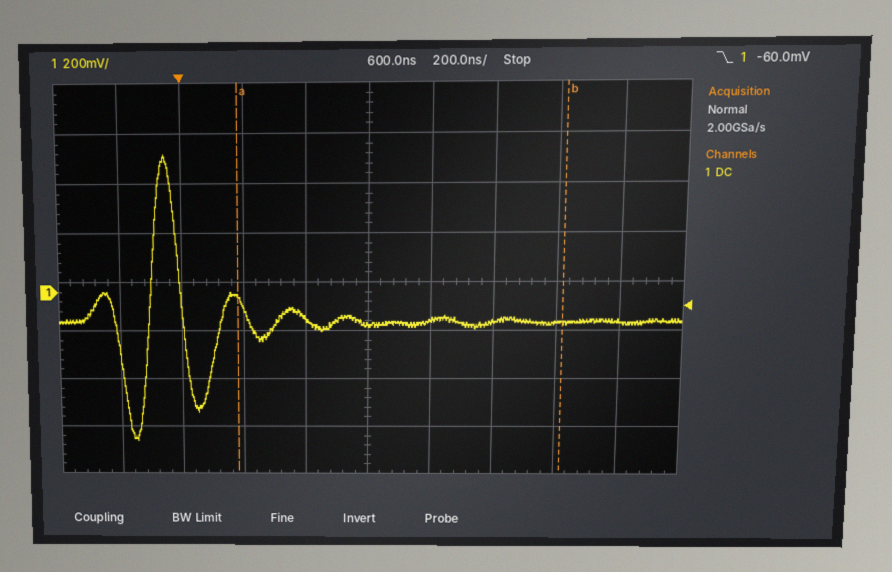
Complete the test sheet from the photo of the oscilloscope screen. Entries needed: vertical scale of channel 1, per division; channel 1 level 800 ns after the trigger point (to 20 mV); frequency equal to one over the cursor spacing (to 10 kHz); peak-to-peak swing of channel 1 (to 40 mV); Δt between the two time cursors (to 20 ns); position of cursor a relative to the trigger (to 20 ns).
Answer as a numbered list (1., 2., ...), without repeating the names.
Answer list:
1. 200 mV
2. -120 mV
3. 960 kHz
4. 1.16 V
5. 1.04 µs
6. +180 ns
